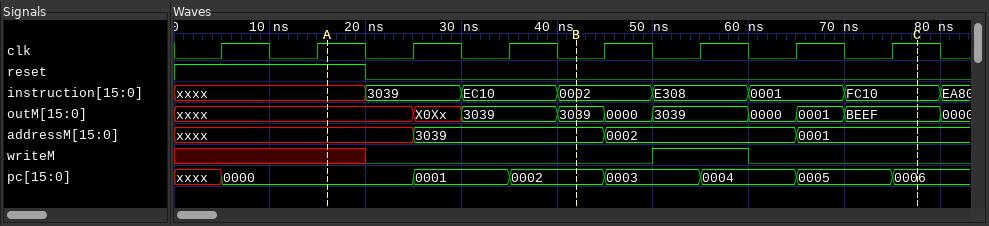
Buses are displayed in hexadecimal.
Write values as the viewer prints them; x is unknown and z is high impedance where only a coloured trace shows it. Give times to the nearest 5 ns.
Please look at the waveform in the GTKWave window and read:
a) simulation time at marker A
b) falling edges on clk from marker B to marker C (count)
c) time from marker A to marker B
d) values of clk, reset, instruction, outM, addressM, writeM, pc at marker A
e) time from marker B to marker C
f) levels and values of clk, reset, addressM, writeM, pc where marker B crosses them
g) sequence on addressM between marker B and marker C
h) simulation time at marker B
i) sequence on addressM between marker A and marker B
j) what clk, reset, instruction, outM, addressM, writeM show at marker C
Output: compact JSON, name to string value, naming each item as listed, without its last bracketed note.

{"simulation time at marker A": "15 ns", "falling edges on clk from marker B to marker C": "3", "time from marker A to marker B": "25 ns", "values of clk, reset, instruction, outM, addressM, writeM, pc at marker A": "clk=1, reset=1, instruction=xxxx, outM=xxxx, addressM=xxxx, writeM=x, pc=0000", "time from marker B to marker C": "35 ns", "levels and values of clk, reset, addressM, writeM, pc where marker B crosses them": "clk=0, reset=0, addressM=3039, writeM=0, pc=0002", "sequence on addressM between marker B and marker C": "3039, 0002, 0001", "simulation time at marker B": "40 ns", "sequence on addressM between marker A and marker B": "xxxx, 3039", "what clk, reset, instruction, outM, addressM, writeM show at marker C": "clk=1, reset=0, instruction=FC10, outM=BEEF, addressM=0001, writeM=0"}
